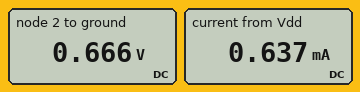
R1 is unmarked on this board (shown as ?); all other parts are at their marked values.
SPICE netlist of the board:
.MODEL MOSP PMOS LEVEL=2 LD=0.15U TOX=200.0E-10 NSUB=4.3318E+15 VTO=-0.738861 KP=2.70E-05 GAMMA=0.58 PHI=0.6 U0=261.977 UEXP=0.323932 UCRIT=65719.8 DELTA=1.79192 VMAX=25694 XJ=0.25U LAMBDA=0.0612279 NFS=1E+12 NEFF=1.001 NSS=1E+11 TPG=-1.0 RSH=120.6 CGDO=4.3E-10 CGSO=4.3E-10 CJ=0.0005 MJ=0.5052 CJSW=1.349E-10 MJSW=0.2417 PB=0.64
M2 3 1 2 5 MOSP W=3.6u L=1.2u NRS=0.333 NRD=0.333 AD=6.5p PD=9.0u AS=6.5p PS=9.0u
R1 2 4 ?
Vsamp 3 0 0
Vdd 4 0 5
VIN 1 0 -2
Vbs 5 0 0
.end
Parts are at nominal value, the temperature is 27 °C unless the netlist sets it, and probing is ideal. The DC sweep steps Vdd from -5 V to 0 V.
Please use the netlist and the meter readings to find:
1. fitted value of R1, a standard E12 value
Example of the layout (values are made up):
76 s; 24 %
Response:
6.8 kΩ
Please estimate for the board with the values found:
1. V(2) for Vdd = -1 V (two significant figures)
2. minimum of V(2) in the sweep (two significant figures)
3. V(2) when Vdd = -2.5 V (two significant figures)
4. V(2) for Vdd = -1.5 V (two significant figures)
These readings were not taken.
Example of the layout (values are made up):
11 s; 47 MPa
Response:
-660 mV; -4.5 V; -2.1 V; -1.1 V
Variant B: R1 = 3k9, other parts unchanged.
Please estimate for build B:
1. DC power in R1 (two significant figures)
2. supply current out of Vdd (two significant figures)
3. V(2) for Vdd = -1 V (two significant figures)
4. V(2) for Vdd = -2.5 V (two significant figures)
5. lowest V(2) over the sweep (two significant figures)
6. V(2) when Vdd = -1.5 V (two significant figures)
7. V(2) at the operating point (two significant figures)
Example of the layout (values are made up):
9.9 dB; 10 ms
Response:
4.7 mW; 1.1 mA; -790 mV; -2.3 V; -4.7 V; -1.3 V; 700 mV
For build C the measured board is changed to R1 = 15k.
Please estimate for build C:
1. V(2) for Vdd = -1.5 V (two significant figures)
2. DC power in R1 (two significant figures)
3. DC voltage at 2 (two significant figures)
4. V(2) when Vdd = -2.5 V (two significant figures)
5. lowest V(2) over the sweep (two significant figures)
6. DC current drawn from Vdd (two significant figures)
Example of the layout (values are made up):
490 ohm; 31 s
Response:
-720 mV; 1.3 mW; 630 mV; -1.6 V; -3.9 V; 290 µA
